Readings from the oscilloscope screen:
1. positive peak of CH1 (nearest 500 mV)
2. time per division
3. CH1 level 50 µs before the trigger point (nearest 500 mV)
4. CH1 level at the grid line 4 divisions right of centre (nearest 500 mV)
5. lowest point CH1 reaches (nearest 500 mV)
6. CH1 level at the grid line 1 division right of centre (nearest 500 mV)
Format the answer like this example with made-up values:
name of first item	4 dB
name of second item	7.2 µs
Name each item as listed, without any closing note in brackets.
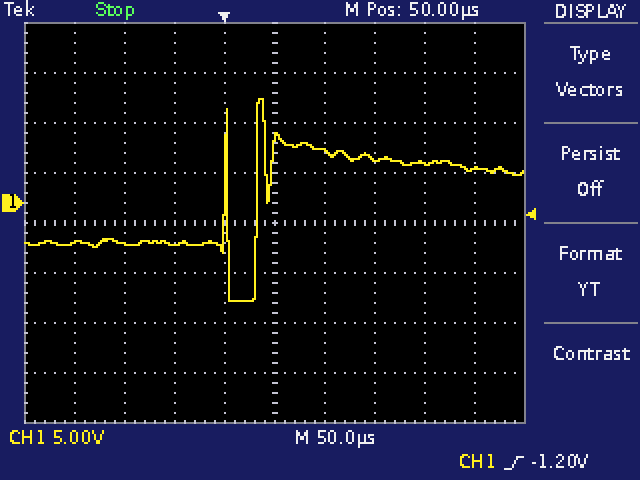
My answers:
positive peak of CH1	10.5 V
time per division	50 µs
CH1 level 50 µs before the trigger point	-4.0 V
CH1 level at the grid line 4 divisions right of centre	3.5 V
lowest point CH1 reaches	-10.0 V
CH1 level at the grid line 1 division right of centre	5.0 V
